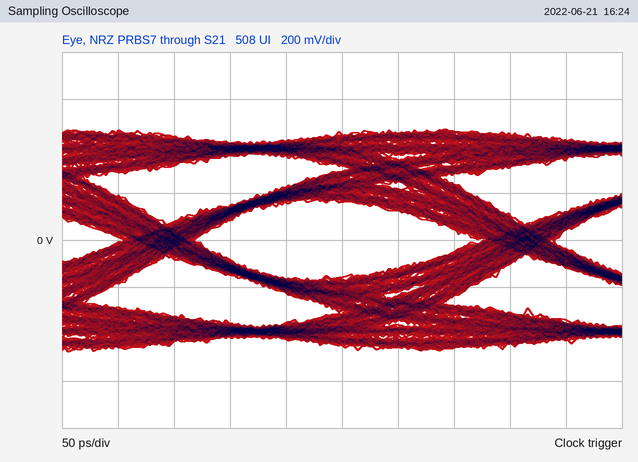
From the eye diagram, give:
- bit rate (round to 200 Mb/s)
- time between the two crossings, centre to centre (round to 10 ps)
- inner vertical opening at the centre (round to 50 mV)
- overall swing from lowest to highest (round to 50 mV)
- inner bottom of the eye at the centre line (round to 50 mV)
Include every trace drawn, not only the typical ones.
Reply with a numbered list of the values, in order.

1. 3.2 Gb/s
2. 320 ps
3. 300 mV
4. 950 mV
5. -150 mV
